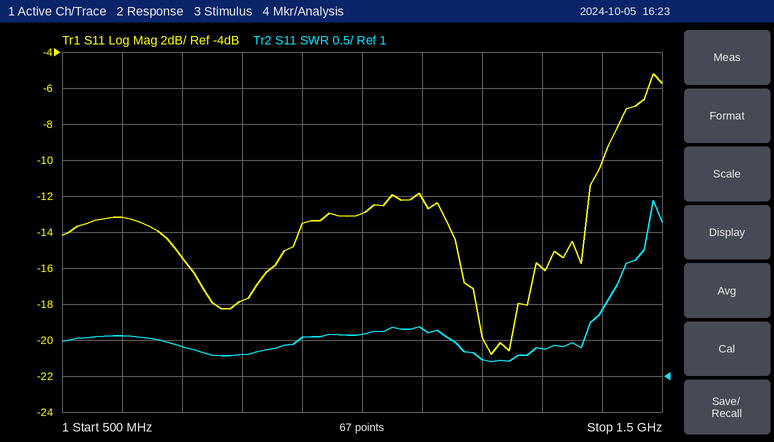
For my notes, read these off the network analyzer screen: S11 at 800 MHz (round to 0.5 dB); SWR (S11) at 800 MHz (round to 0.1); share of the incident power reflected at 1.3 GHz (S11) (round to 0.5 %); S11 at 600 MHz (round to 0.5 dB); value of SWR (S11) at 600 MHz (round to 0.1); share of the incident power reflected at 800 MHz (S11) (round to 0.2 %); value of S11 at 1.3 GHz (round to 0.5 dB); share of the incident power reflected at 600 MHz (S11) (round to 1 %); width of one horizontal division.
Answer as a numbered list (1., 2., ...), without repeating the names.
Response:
1. -18.0 dB
2. 1.3
3. 2.5 %
4. -13.0 dB
5. 1.6
6. 1.6 %
7. -16.0 dB
8. 5 %
9. 100 MHz
